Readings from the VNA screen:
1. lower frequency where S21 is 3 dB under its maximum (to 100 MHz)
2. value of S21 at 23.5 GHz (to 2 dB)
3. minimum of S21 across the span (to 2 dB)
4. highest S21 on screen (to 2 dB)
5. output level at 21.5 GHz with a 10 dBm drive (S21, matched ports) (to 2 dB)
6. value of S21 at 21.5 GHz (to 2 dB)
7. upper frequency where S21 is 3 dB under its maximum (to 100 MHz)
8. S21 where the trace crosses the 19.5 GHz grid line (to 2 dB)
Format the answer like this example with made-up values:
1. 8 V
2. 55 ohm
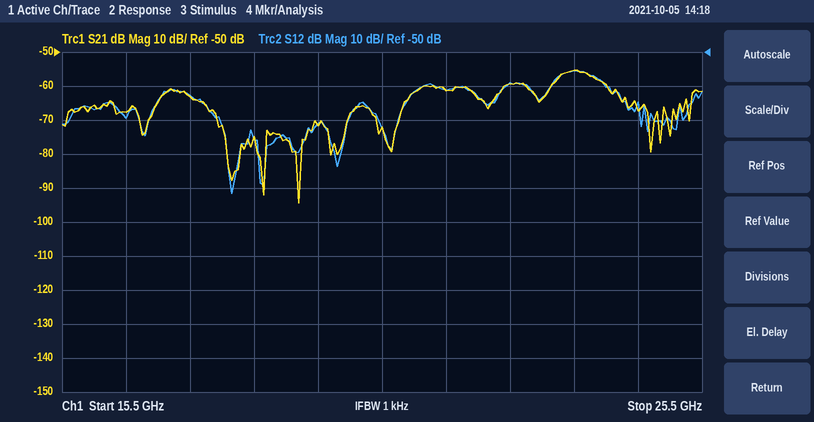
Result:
1. 23.2 GHz
2. -56 dB
3. -94 dB
4. -56 dB
5. -52 dBm
6. -62 dB
7. 23.9 GHz
8. -72 dB
